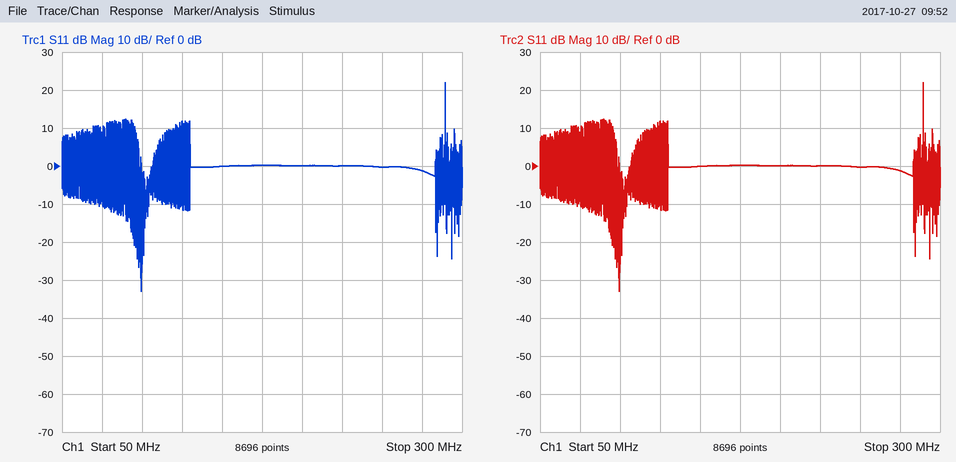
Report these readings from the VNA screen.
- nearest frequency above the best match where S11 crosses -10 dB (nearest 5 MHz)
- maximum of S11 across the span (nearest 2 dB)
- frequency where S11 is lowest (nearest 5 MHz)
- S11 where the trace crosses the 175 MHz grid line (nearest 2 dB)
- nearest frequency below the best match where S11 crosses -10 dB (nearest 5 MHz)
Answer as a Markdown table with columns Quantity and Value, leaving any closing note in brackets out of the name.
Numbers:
| Quantity | Value |
|---|---|
| nearest frequency above the best match where S11 crosses -10 dB | 100 MHz |
| maximum of S11 across the span | 22 dB |
| frequency where S11 is lowest | 100 MHz |
| S11 where the trace crosses the 175 MHz grid line | 0 dB |
| nearest frequency below the best match where S11 crosses -10 dB | 100 MHz |
